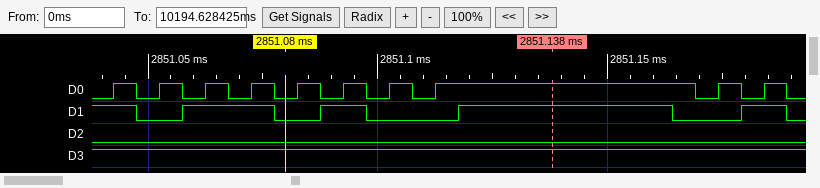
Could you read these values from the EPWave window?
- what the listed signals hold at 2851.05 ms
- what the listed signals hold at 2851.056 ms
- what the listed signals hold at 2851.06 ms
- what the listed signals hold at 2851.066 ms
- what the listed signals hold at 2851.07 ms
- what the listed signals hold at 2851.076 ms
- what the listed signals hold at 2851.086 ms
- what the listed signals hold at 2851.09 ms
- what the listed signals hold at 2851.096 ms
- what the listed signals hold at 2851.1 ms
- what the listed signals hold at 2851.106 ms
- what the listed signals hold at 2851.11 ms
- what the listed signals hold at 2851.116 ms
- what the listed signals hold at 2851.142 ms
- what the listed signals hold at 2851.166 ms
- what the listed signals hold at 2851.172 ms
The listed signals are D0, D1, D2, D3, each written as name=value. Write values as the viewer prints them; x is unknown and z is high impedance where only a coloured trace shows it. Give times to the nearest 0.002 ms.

D0=0, D1=0, D2=0, D3=1
D0=1, D1=0, D2=0, D3=1
D0=0, D1=1, D2=0, D3=1
D0=1, D1=1, D2=0, D3=1
D0=0, D1=1, D2=0, D3=1
D0=1, D1=1, D2=0, D3=1
D0=1, D1=0, D2=0, D3=1
D0=0, D1=1, D2=0, D3=1
D0=1, D1=1, D2=0, D3=1
D0=0, D1=0, D2=0, D3=1
D0=1, D1=0, D2=0, D3=1
D0=0, D1=0, D2=0, D3=1
D0=1, D1=0, D2=0, D3=1
D0=1, D1=1, D2=0, D3=1
D0=1, D1=0, D2=0, D3=1
D0=0, D1=0, D2=0, D3=1
